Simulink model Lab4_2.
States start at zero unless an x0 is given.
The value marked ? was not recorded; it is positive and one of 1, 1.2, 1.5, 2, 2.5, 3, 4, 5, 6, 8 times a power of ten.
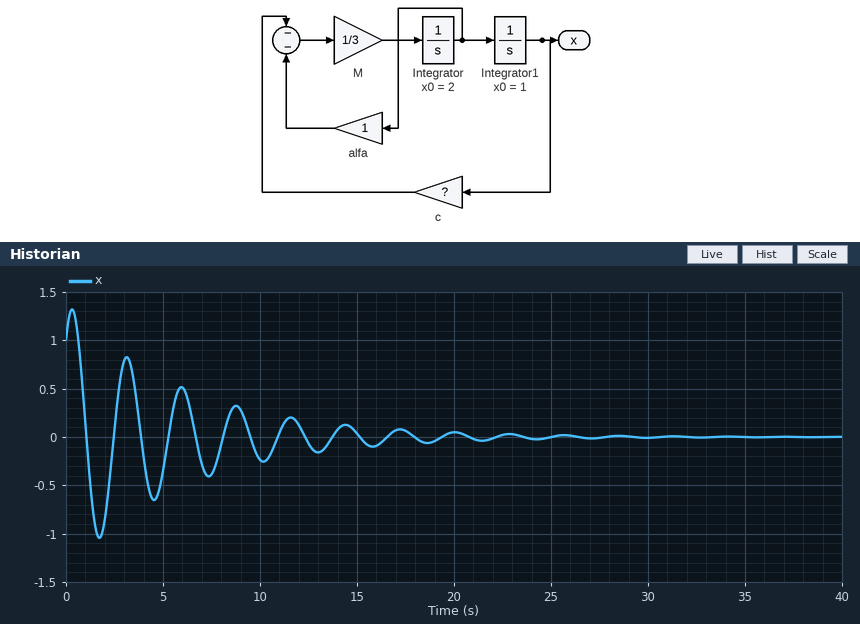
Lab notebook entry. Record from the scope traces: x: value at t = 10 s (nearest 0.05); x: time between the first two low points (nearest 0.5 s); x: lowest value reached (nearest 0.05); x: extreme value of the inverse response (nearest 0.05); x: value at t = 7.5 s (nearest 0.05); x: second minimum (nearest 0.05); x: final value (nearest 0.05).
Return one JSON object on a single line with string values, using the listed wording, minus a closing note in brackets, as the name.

{"x: value at t = 10 s": "-0.25", "x: time between the first two low points": "3.0 s", "x: lowest value reached": "-1.05", "x: extreme value of the inverse response": "1.30", "x: value at t = 7.5 s": "-0.40", "x: second minimum": "-0.65", "x: final value": "0.00"}
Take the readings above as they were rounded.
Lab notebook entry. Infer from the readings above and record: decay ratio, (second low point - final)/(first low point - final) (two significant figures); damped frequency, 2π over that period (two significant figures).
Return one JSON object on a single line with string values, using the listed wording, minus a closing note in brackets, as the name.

{"decay ratio, (second low point - final)/(first low point - final)": "0.62", "damped frequency, 2π over that period": "2.1 rad/s"}
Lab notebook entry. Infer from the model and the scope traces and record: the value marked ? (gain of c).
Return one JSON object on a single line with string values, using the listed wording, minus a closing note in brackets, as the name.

{"the value marked ?": "15"}
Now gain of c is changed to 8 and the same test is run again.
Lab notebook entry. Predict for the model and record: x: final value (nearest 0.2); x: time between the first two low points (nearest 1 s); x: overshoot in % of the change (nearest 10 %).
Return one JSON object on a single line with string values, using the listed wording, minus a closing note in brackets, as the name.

{"x: final value": "0.0", "x: time between the first two low points": "4 s", "x: overshoot in % of the change": "110 %"}
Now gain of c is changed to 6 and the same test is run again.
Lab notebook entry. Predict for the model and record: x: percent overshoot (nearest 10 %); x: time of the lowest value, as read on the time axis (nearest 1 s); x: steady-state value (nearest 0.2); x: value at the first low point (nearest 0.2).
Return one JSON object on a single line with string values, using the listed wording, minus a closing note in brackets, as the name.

{"x: percent overshoot": "110 %", "x: time of the lowest value, as read on the time axis": "3 s", "x: steady-state value": "0.0", "x: value at the first low point": "-1.2"}
